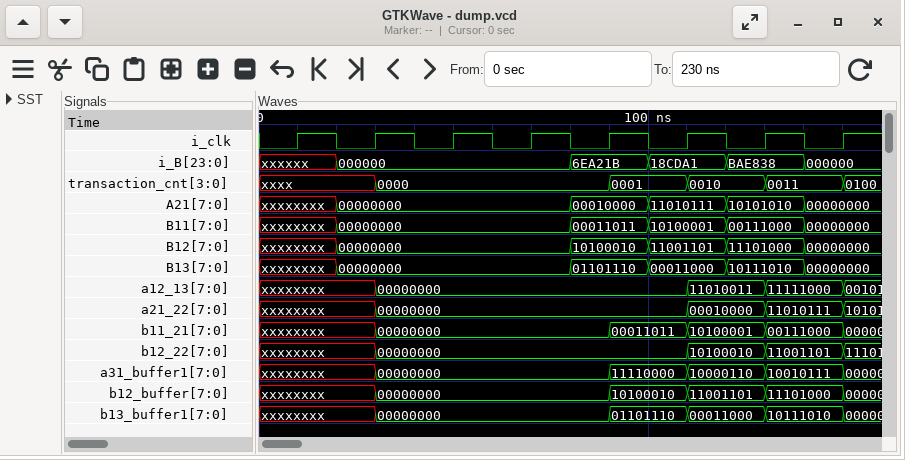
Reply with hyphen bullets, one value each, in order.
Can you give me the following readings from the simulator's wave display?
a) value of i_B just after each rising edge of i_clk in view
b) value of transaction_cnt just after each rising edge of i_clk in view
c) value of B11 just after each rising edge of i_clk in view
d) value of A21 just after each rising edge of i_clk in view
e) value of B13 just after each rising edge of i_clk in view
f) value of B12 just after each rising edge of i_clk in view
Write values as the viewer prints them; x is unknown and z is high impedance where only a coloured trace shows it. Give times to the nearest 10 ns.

- xxxxxx, 000000, 000000, 000000, 6EA21B, 18CDA1, BAE838, 000000
- xxxx, 0000, 0000, 0000, 0001, 0010, 0011, 0100
- xxxxxxxx, 00000000, 00000000, 00000000, 00011011, 10100001, 00111000, 00000000
- xxxxxxxx, 00000000, 00000000, 00000000, 00010000, 11010111, 10101010, 00000000
- xxxxxxxx, 00000000, 00000000, 00000000, 01101110, 00011000, 10111010, 00000000
- xxxxxxxx, 00000000, 00000000, 00000000, 10100010, 11001101, 11101000, 00000000
